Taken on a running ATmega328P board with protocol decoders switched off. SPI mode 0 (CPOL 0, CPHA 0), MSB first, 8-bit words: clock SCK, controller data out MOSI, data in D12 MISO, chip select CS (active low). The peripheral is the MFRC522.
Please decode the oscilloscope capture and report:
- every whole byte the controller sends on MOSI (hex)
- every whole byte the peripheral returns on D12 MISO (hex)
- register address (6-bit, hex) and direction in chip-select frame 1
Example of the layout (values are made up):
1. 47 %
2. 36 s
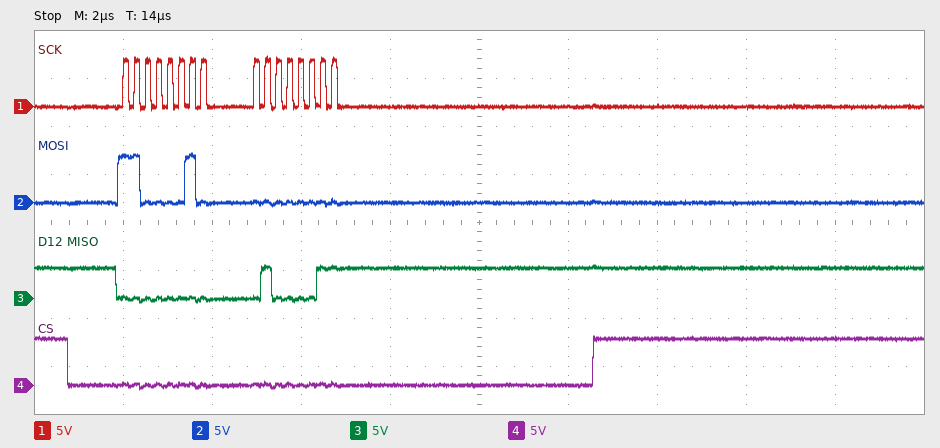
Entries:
1. C2 00
2. 00 43
3. 0x21 read
